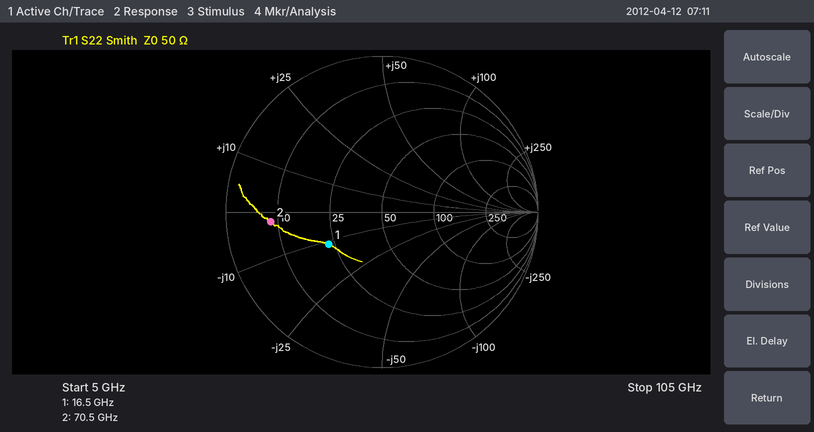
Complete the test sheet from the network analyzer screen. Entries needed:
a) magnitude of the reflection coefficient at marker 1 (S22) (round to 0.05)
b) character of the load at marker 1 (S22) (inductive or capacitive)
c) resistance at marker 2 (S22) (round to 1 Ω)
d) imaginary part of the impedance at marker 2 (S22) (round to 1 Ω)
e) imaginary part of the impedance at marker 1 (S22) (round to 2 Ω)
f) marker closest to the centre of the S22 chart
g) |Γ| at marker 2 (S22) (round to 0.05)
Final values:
0.40
capacitive
8 Ω
-2 Ω
-12 Ω
marker 1
0.70
